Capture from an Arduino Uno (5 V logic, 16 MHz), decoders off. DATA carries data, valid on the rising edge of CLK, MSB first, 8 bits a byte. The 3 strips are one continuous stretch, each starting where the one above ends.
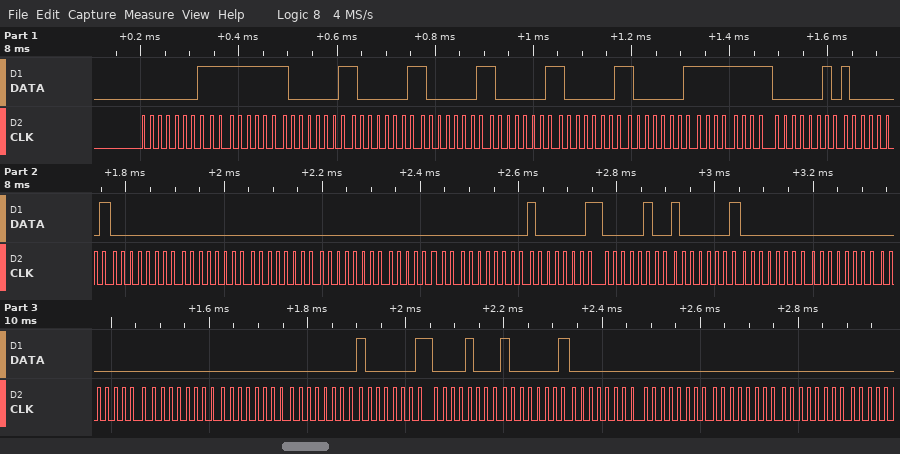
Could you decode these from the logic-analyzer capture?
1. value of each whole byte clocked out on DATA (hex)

01 FF 81 81 81 81 81 81 FF 02 81 00 00 00 00 00 00 81 04 81 00 00 00 00 00 00 81 08 81 00 00 00 00
